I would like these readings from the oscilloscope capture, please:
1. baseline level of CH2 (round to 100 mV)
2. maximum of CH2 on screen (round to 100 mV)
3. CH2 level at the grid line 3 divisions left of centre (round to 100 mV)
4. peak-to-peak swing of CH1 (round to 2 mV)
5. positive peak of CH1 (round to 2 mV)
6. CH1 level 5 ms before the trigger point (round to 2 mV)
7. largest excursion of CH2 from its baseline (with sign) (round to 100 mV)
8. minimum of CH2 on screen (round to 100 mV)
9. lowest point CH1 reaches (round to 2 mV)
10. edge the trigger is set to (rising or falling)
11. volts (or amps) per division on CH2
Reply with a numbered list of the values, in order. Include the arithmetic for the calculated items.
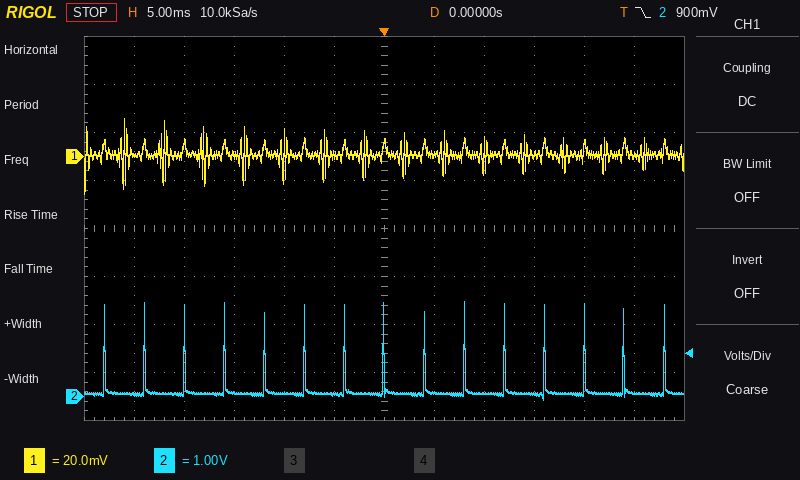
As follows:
1. 100 mV
2. 2.0 V
3. 100 mV
4. 16 mV − (-16 mV) = 32 mV
5. 16 mV
6. 0 mV
7. 2.0 V − (100 mV) = +1.9 V
8. -100 mV
9. -16 mV
10. falling
11. 1 V
